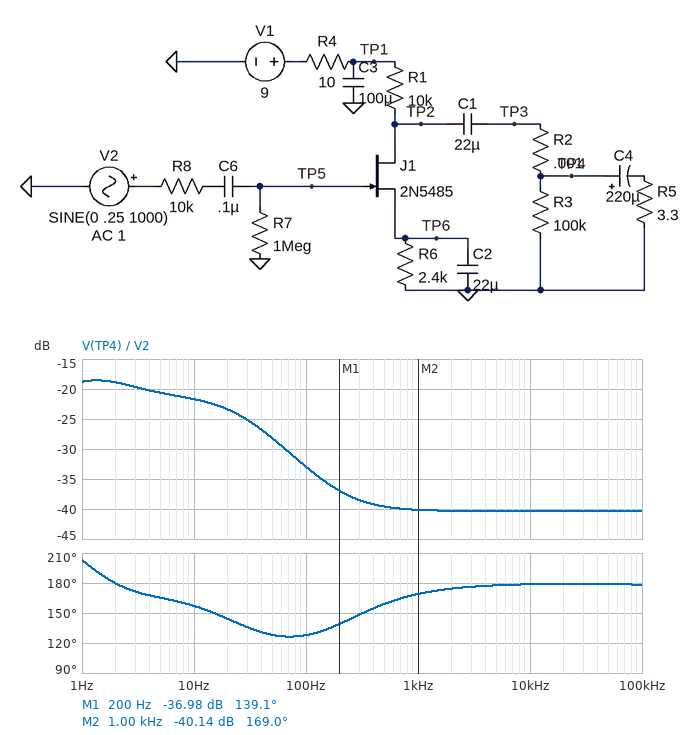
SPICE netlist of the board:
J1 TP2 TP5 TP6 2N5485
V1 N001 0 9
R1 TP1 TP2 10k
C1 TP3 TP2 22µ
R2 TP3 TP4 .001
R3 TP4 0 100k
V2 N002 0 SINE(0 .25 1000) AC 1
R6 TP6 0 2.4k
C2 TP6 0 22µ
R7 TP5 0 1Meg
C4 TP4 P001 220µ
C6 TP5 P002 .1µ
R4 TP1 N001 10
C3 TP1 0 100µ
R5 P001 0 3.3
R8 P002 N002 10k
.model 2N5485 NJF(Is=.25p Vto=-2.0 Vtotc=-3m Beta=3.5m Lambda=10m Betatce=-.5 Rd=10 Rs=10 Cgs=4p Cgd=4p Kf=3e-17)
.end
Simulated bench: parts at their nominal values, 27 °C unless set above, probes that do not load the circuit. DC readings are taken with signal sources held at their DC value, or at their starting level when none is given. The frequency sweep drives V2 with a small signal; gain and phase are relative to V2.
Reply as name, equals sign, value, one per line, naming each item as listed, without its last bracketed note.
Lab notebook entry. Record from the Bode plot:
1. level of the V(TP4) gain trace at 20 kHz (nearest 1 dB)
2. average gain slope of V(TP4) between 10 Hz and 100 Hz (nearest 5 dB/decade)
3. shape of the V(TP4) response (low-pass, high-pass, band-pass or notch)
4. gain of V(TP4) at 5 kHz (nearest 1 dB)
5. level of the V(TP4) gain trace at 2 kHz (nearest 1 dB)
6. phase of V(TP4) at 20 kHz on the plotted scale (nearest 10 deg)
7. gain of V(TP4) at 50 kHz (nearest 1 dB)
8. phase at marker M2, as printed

level of the V(TP4) gain trace at 20 kHz = -40 dB
average gain slope of V(TP4) between 10 Hz and 100 Hz = -10 dB/decade
shape of the V(TP4) response = low-pass
gain of V(TP4) at 5 kHz = -40 dB
level of the V(TP4) gain trace at 2 kHz = -40 dB
phase of V(TP4) at 20 kHz on the plotted scale = 180 deg
gain of V(TP4) at 50 kHz = -40 dB
phase at marker M2, as printed = 169.0 deg
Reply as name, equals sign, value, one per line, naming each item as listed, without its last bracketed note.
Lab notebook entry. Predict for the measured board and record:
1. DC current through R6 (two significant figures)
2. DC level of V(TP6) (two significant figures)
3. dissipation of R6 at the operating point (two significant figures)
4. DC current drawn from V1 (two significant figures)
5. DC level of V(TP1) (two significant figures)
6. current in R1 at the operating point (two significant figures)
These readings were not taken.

DC current through R6 = 650 µA
DC level of V(TP6) = 1.6 V
dissipation of R6 at the operating point = 1.0 mW
DC current drawn from V1 = 650 µA
DC level of V(TP1) = 9.0 V
current in R1 at the operating point = 650 µA
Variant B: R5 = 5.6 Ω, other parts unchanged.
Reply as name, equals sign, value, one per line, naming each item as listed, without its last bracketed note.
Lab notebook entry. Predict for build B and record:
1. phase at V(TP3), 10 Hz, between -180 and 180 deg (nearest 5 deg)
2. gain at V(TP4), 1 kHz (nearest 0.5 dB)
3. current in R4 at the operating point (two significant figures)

phase at V(TP3), 10 Hz, between -180 and 180 deg = 160 deg
gain at V(TP4), 1 kHz = -35.5 dB
current in R4 at the operating point = 650 µA
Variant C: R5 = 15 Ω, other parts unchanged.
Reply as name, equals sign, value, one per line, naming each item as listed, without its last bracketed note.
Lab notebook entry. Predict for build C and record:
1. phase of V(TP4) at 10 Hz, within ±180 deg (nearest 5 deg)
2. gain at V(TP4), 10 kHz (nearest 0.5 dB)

phase of V(TP4) at 10 Hz, within ±180 deg = 165 deg
gain at V(TP4), 10 kHz = -27.0 dB
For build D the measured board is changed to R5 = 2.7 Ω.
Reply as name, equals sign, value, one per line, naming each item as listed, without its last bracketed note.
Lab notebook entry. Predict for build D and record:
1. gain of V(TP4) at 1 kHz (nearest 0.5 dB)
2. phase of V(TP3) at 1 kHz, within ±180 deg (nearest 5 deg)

gain of V(TP4) at 1 kHz = -42.0 dB
phase of V(TP3) at 1 kHz, within ±180 deg = 165 deg
